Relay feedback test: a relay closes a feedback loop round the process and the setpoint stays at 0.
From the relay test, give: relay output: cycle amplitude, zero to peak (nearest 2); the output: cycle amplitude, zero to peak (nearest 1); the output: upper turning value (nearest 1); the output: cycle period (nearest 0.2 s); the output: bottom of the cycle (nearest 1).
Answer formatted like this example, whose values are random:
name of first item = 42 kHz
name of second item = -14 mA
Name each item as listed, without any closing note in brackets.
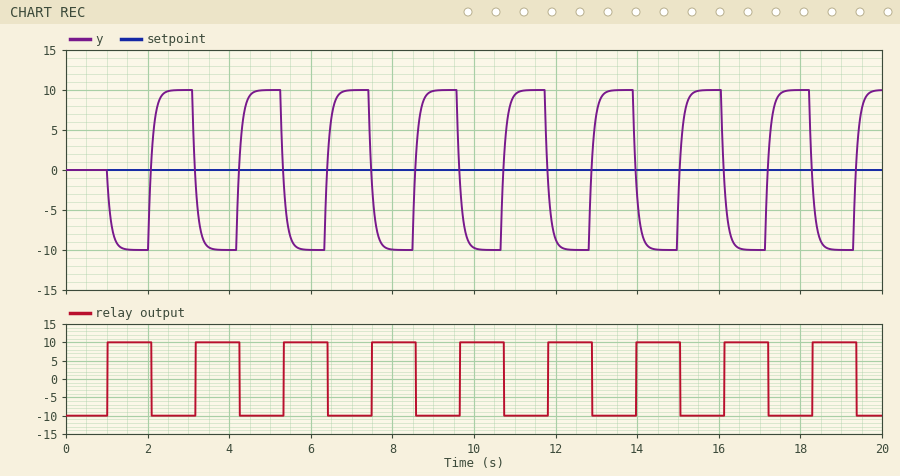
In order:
relay output: cycle amplitude, zero to peak = 10
the output: cycle amplitude, zero to peak = 10
the output: upper turning value = 10
the output: cycle period = 2.2 s
the output: bottom of the cycle = -10
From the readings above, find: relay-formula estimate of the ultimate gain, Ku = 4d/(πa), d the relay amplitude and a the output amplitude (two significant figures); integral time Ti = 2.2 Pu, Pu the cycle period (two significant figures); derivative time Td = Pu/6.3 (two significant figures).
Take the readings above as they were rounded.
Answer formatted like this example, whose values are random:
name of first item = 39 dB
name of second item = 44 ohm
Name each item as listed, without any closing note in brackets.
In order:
relay-formula estimate of the ultimate gain, Ku = 4d/(πa), d the relay amplitude and a the output amplitude = 1.3
integral time Ti = 2.2 Pu, Pu the cycle period = 4.8 s
derivative time Td = Pu/6.3 = 0.35 s
